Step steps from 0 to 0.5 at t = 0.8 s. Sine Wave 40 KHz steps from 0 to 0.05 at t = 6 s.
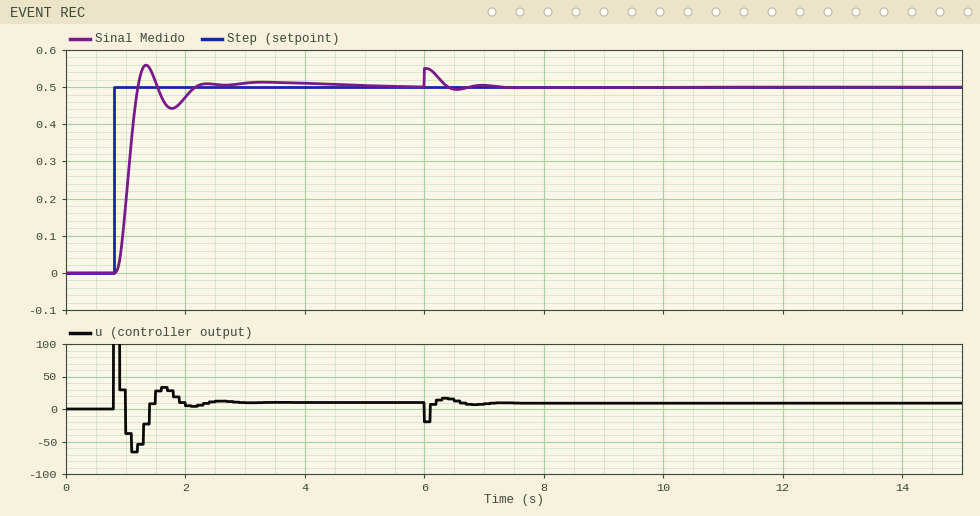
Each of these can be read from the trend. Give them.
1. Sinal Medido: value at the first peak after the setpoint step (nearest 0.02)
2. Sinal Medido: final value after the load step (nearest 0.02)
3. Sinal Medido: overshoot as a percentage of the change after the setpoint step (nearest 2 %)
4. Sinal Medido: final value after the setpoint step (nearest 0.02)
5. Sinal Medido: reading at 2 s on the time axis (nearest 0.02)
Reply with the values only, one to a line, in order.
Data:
0.56
0.50
12 %
0.50
0.48
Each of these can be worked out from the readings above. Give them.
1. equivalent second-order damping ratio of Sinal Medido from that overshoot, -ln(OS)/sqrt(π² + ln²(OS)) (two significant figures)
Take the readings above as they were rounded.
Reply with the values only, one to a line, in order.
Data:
0.56
